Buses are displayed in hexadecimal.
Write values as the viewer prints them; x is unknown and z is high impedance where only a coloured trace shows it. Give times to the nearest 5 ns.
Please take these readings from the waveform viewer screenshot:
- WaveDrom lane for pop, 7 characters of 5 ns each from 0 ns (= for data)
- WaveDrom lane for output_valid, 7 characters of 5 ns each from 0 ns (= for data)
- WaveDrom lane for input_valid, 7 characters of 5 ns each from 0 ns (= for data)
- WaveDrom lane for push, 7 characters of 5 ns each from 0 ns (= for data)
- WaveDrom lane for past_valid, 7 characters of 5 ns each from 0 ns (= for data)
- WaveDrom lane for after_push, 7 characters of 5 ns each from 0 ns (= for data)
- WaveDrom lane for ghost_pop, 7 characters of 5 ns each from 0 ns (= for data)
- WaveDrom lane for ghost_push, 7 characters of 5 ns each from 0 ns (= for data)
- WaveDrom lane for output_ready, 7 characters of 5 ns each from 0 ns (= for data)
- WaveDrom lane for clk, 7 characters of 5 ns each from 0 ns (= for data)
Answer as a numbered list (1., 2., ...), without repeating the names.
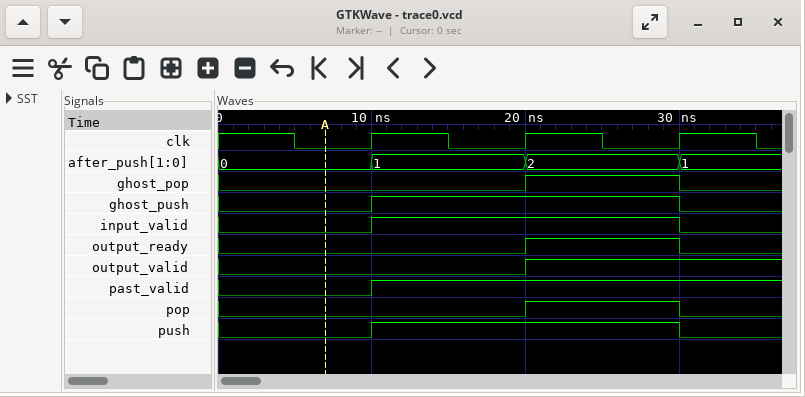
1. {name: 'pop', wave: '0...1.0'}
2. {name: 'output_valid', wave: '0...1..'}
3. {name: 'input_valid', wave: '0.1...0'}
4. {name: 'push', wave: '0.1...0'}
5. {name: 'past_valid', wave: '0.1....'}
6. {name: 'after_push', wave: '=.=.=.=', data: '0 1 2 1'}
7. {name: 'ghost_pop', wave: '0...1.0'}
8. {name: 'ghost_push', wave: '0.1...0'}
9. {name: 'output_ready', wave: '0...1.0'}
10. {name: 'clk', wave: '1010101'}
